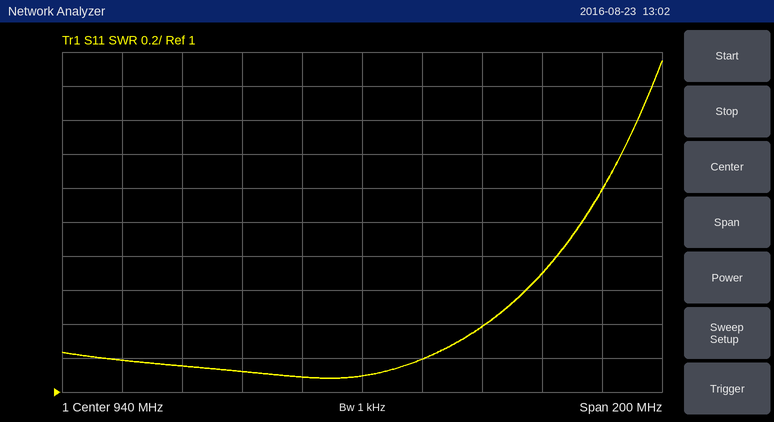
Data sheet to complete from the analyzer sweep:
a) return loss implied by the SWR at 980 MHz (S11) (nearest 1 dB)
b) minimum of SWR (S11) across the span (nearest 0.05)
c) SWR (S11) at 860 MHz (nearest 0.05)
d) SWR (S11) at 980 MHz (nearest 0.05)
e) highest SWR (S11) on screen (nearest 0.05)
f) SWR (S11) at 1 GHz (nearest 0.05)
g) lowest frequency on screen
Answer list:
16 dB
1.10
1.20
1.40
2.95
1.70
840 MHz
